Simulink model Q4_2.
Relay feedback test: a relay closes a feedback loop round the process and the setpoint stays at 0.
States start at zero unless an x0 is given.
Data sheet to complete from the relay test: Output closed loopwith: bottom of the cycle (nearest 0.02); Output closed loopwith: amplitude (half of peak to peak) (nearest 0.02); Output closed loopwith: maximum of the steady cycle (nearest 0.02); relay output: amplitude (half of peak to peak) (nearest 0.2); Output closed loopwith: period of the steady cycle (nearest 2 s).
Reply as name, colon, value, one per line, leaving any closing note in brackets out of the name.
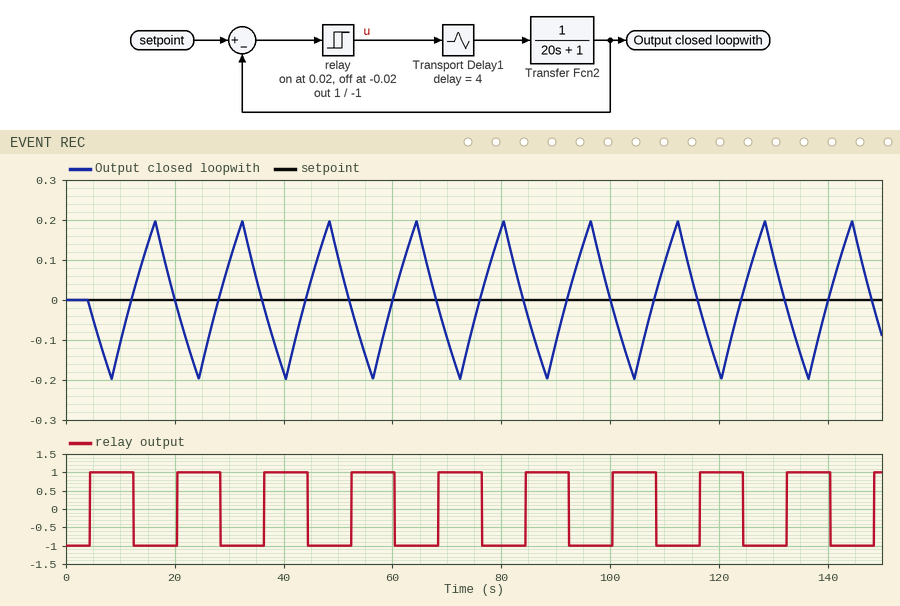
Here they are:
Output closed loopwith: bottom of the cycle: -0.20
Output closed loopwith: amplitude (half of peak to peak): 0.20
Output closed loopwith: maximum of the steady cycle: 0.20
relay output: amplitude (half of peak to peak): 1.0
Output closed loopwith: period of the steady cycle: 16 s
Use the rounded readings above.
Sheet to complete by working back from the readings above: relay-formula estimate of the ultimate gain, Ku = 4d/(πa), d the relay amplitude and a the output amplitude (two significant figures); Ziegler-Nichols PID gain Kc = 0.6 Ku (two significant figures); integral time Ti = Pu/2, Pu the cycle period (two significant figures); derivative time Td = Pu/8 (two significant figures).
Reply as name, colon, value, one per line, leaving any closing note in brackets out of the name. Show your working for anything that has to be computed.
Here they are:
relay-formula estimate of the ultimate gain, Ku = 4d/(πa), d the relay amplitude and a the output amplitude: 4 × 1 / (π × 0.2) = 6.4
Ziegler-Nichols PID gain Kc = 0.6 Ku: 0.6 × 6.4 = 3.8
integral time Ti = Pu/2, Pu the cycle period: 16 / 2 = 8.0 s
derivative time Td = Pu/8: 16 / 8 = 2.0 s
